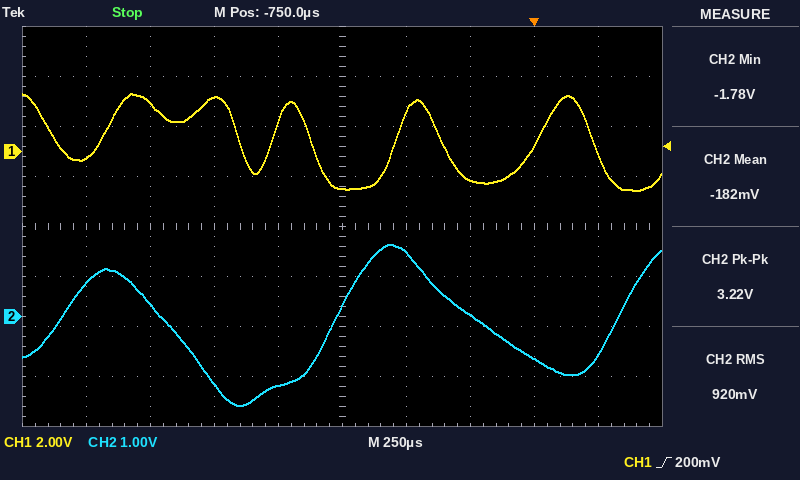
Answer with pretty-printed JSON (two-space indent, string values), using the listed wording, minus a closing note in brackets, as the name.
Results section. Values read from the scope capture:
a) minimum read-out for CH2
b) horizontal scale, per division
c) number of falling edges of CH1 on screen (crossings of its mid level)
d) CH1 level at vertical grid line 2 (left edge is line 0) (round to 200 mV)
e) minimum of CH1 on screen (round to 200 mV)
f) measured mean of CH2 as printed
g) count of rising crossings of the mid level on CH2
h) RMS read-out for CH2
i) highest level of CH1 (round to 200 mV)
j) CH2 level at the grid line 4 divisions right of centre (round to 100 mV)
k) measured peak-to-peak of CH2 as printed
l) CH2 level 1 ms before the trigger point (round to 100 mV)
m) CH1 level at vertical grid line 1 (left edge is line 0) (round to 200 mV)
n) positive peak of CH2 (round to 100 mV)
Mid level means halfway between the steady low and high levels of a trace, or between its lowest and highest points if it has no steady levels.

{
  "minimum read-out for CH2": "-1.78 V",
  "horizontal scale, per division": "250 µs",
  "number of falling edges of CH1 on screen": "5",
  "CH1 level at vertical grid line 2 (left edge is line 0)": "2.0 V",
  "minimum of CH1 on screen": "-1.6 V",
  "measured mean of CH2 as printed": "-182 mV",
  "count of rising crossings of the mid level on CH2": "3",
  "RMS read-out for CH2": "920 mV",
  "highest level of CH1": "2.4 V",
  "CH2 level at the grid line 4 divisions right of centre": "-800 mV",
  "measured peak-to-peak of CH2 as printed": "3.22 V",
  "CH2 level 1 ms before the trigger point": "-1.4 V",
  "CH1 level at vertical grid line 1 (left edge is line 0)": "-200 mV",
  "positive peak of CH2": "1.4 V"
}
